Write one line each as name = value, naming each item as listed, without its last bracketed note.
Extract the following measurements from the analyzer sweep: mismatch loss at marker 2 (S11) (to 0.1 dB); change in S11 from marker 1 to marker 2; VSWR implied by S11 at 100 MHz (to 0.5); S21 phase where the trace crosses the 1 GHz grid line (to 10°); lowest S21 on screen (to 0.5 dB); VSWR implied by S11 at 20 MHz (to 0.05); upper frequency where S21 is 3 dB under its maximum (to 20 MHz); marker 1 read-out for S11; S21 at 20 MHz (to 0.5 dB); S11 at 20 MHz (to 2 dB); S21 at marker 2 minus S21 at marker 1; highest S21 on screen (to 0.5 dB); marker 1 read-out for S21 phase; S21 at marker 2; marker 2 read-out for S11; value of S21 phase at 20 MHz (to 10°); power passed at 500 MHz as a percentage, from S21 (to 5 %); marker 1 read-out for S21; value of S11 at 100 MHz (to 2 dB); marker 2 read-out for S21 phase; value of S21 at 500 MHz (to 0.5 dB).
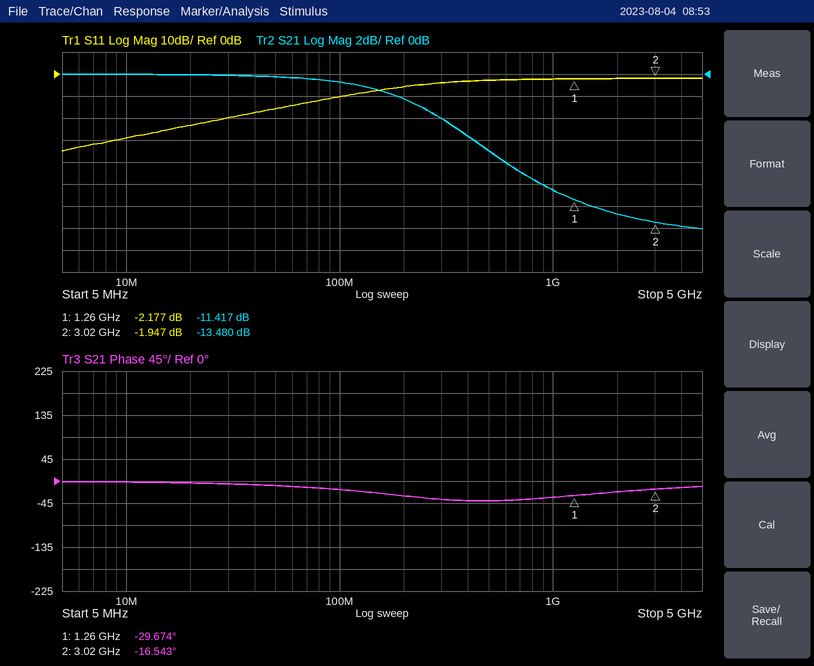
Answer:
mismatch loss at marker 2 (S11) = 4.4 dB
change in S11 from marker 1 to marker 2 = 0.230 dB
VSWR implied by S11 at 100 MHz = 2.0
S21 phase where the trace crosses the 1 GHz grid line = -30°
lowest S21 on screen = -14.0 dB
VSWR implied by S11 at 20 MHz = 1.15
upper frequency where S21 is 3 dB under its maximum = 240 MHz
marker 1 read-out for S11 = -2.177 dB
S21 at 20 MHz = 0.0 dB
S11 at 20 MHz = -24 dB
S21 at marker 2 minus S21 at marker 1 = -2.063 dB
highest S21 on screen = 0.0 dB
marker 1 read-out for S21 phase = -29.674°
S21 at marker 2 = -13.480 dB
marker 2 read-out for S11 = -1.947 dB
value of S21 phase at 20 MHz = 0°
power passed at 500 MHz as a percentage, from S21 = 20 %
marker 1 read-out for S21 = -11.417 dB
value of S11 at 100 MHz = -10 dB
marker 2 read-out for S21 phase = -16.543°
value of S21 at 500 MHz = -7.0 dB
